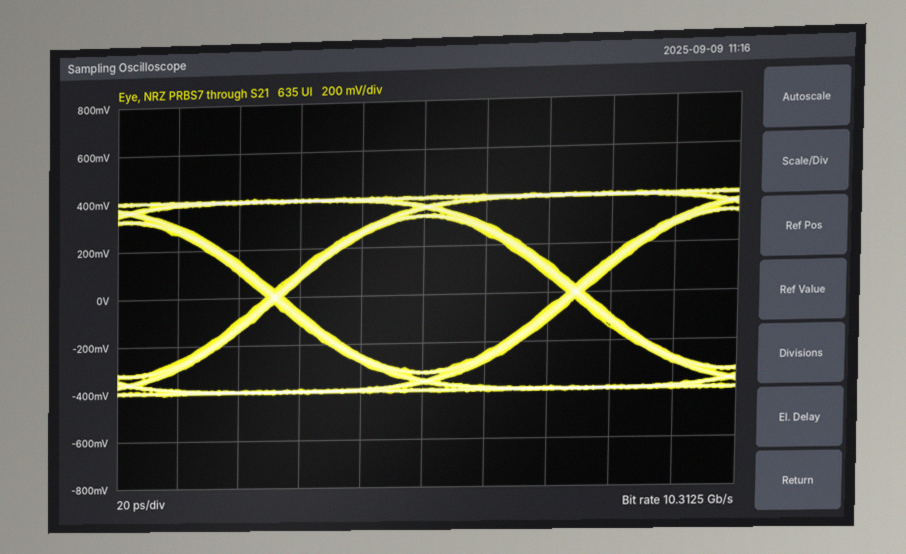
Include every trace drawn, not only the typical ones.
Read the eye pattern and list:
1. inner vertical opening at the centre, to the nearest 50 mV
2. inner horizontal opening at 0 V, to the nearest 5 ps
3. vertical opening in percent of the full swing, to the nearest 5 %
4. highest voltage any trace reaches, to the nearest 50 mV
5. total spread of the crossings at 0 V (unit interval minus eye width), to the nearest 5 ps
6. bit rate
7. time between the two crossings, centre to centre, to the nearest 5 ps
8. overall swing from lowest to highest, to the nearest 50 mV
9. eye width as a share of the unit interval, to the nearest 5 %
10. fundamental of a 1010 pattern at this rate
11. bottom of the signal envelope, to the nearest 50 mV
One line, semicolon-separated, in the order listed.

650 mV; 90 ps; 80 %; 400 mV; 5 ps; 10.3125 Gb/s; 95 ps; 800 mV; 95 %; 5.15625 GHz; -400 mV
